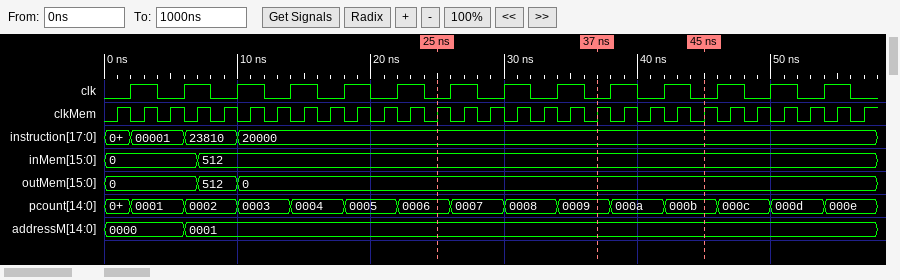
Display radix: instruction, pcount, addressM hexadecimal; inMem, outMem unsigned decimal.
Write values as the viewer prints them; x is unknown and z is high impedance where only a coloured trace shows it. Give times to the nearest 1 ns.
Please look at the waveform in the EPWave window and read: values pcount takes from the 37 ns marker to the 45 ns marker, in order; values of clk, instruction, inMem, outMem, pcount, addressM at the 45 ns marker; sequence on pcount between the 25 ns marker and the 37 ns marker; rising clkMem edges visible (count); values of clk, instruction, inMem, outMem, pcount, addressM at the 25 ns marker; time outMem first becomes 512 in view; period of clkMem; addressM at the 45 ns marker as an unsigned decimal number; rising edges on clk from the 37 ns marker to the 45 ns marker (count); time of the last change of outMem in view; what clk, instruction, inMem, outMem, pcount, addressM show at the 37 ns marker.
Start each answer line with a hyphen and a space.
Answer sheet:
- 0009, 000a, 000b
- clk=0, instruction=20000, inMem=512, outMem=0, pcount=000b, addressM=0001
- 0006, 0007, 0008, 0009
- 29
- clk=0, instruction=20000, inMem=512, outMem=0, pcount=0006, addressM=0001
- 7 ns
- 2 ns
- 1
- 2
- 10 ns
- clk=0, instruction=20000, inMem=512, outMem=0, pcount=0009, addressM=0001
